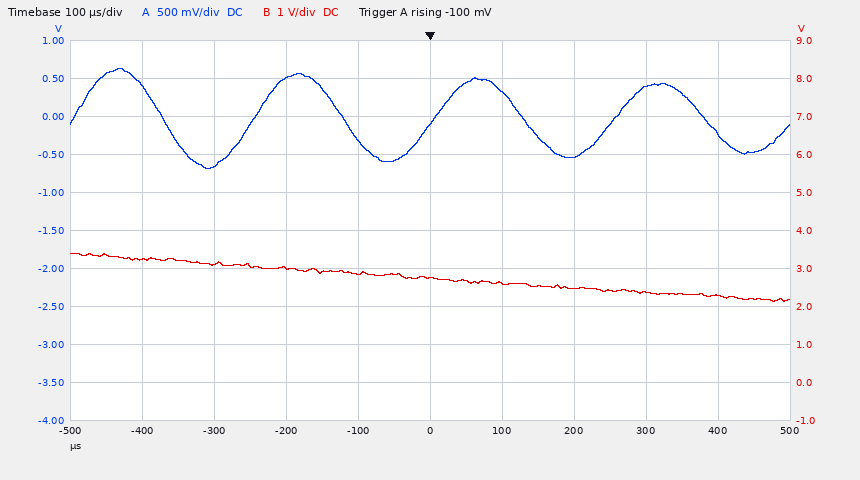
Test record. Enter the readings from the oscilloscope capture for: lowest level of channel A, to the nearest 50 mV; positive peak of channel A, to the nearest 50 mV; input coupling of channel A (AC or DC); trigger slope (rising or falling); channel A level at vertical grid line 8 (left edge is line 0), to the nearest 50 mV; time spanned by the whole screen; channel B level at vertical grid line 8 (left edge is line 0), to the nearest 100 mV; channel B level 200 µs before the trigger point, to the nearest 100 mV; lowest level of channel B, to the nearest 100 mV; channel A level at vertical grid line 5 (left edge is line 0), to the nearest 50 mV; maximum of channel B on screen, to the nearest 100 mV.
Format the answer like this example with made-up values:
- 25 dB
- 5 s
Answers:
- -700 mV
- 650 mV
- DC
- rising
- 400 mV
- 1 ms
- 2.4 V
- 3.0 V
- 2.1 V
- -100 mV
- 3.4 V
